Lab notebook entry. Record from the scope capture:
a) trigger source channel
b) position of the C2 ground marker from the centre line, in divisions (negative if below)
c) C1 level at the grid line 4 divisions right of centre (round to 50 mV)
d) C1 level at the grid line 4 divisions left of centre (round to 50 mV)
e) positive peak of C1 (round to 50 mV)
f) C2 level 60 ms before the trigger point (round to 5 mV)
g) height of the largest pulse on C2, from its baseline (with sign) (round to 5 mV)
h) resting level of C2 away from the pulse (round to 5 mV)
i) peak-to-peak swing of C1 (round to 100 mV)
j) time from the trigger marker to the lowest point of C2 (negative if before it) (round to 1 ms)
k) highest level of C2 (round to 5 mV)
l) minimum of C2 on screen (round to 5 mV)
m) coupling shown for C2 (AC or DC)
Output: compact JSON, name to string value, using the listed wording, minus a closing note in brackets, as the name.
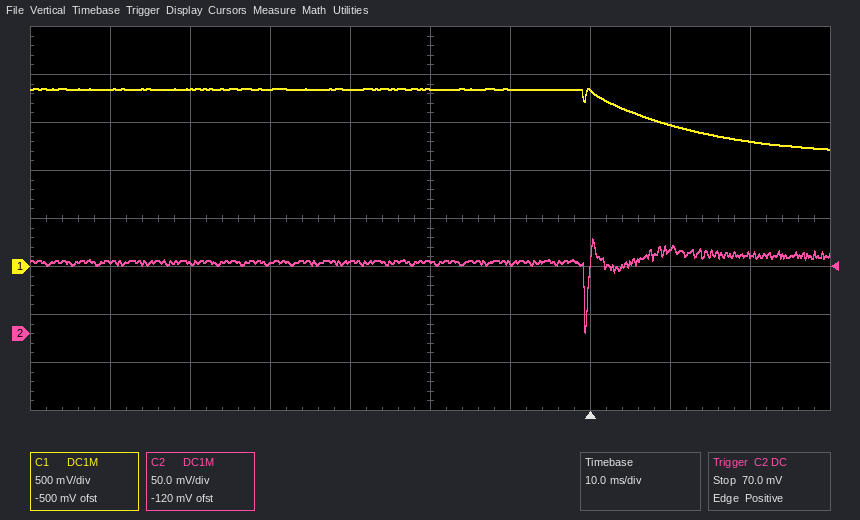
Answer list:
{"trigger source channel": "C2", "position of the C2 ground marker from the centre line, in divisions": "-2.4 div", "C1 level at the grid line 4 divisions right of centre": "1.30 V", "C1 level at the grid line 4 divisions left of centre": "1.85 V", "positive peak of C1": "1.85 V", "C2 level 60 ms before the trigger point": "75 mV", "height of the largest pulse on C2, from its baseline (with sign)": "-75 mV", "resting level of C2 away from the pulse": "75 mV", "peak-to-peak swing of C1": "600 mV", "time from the trigger marker to the lowest point of C2 (negative if before it)": "-1 ms", "highest level of C2": "100 mV", "minimum of C2 on screen": "0 mV", "coupling shown for C2": "DC"}
